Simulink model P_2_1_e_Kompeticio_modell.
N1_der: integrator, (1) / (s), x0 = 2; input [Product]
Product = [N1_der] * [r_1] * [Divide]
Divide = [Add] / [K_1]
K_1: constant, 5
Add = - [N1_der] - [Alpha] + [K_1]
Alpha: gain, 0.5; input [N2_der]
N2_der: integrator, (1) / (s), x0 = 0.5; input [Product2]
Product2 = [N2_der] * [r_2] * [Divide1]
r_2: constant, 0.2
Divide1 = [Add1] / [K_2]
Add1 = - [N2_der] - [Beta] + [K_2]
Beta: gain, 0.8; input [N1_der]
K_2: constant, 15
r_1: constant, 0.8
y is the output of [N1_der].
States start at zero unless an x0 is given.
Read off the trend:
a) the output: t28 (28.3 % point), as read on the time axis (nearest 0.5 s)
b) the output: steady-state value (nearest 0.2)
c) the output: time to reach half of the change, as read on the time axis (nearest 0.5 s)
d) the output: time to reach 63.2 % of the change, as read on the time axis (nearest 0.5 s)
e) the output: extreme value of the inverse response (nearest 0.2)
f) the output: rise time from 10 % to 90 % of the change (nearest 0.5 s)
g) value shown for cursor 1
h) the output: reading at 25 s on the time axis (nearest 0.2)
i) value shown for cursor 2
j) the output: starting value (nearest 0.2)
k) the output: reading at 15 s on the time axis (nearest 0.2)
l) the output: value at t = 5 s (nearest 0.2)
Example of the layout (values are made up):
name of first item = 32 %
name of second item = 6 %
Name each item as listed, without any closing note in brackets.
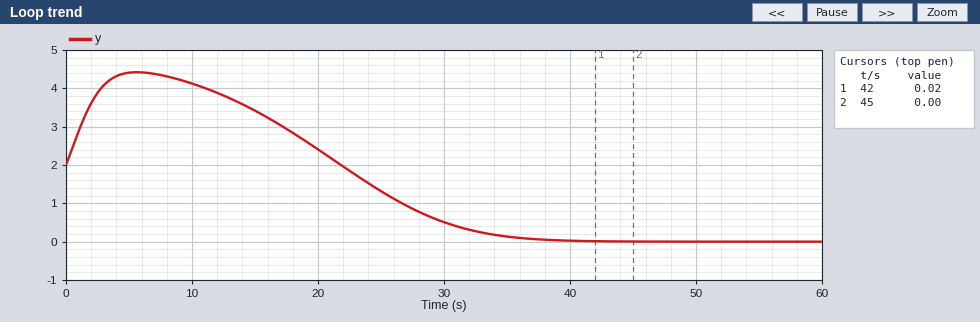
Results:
the output: t28 (28.3 % point), as read on the time axis = 24.5 s
the output: steady-state value = 0.0
the output: time to reach half of the change, as read on the time axis = 26.5 s
the output: time to reach 63.2 % of the change, as read on the time axis = 28.5 s
the output: extreme value of the inverse response = 4.4
the output: rise time from 10 % to 90 % of the change = 11.0 s
value shown for cursor 1 = 0.02
the output: reading at 25 s on the time axis = 1.4
value shown for cursor 2 = 0.00
the output: starting value = 2.0
the output: reading at 15 s on the time axis = 3.4
the output: value at t = 5 s = 4.4
